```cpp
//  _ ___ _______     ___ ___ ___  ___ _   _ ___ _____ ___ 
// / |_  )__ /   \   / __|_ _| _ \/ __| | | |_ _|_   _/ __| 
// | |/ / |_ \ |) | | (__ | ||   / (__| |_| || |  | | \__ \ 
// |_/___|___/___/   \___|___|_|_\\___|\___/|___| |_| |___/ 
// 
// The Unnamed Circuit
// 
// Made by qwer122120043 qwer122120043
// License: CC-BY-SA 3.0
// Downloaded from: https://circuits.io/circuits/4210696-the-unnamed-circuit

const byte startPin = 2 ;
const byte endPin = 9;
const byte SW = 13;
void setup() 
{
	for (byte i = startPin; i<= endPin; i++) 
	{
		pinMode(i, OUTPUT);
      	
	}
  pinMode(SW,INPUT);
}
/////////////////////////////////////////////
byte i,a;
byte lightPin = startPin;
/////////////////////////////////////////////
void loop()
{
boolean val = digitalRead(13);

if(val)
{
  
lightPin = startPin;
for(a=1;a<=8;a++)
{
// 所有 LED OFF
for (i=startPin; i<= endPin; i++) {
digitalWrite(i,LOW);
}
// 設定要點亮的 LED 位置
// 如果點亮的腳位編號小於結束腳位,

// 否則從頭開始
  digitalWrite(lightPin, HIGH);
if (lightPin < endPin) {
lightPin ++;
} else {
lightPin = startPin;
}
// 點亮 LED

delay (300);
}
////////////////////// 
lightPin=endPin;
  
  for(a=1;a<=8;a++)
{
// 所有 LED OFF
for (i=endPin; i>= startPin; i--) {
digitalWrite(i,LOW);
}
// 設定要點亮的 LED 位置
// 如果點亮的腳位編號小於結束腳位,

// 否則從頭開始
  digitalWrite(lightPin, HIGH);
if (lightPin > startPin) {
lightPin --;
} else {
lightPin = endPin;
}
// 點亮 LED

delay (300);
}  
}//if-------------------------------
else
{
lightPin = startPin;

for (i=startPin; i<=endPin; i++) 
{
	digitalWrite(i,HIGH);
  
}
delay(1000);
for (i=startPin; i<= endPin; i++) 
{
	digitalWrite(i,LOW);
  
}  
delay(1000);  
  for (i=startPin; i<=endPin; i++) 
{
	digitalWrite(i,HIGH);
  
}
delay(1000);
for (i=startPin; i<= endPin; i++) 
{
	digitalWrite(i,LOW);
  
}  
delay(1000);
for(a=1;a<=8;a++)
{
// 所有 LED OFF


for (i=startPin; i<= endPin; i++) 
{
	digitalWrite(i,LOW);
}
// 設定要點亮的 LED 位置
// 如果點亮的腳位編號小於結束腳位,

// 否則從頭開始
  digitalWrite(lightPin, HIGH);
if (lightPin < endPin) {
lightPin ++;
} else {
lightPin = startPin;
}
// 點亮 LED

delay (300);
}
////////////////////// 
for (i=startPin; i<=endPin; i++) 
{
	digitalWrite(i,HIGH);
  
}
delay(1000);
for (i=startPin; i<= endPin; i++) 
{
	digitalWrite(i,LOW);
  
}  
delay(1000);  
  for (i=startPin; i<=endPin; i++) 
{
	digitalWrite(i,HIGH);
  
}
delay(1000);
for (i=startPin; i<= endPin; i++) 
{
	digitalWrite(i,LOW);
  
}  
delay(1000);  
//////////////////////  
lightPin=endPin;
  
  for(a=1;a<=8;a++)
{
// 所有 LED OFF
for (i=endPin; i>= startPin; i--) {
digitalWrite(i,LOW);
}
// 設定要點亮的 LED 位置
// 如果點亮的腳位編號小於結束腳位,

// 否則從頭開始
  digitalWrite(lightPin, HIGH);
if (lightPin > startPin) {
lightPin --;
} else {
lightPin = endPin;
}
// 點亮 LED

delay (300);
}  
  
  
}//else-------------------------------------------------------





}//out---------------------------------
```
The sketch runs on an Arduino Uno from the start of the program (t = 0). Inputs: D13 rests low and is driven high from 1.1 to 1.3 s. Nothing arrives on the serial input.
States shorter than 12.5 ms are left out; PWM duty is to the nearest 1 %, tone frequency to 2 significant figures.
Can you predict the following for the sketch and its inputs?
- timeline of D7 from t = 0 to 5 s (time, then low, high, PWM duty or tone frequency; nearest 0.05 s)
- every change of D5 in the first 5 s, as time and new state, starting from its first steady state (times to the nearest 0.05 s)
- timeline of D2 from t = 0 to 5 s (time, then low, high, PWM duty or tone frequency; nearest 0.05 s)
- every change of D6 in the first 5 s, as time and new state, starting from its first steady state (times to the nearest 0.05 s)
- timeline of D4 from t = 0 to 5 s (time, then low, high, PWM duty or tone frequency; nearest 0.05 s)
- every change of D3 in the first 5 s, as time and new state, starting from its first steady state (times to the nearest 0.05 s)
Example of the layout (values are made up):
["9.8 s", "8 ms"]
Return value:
["0 s high; 1 s low; 2 s high; 3 s low", "0 s high; 1 s low; 2 s high; 3 s low; 4.9 s high", "0 s high; 1 s low; 2 s high; 3 s low; 4 s high; 4.3 s low", "0 s high; 1 s low; 2 s high; 3 s low", "0 s high; 1 s low; 2 s high; 3 s low; 4.6 s high; 4.9 s low", "0 s high; 1 s low; 2 s high; 3 s low; 4.3 s high; 4.6 s low"]
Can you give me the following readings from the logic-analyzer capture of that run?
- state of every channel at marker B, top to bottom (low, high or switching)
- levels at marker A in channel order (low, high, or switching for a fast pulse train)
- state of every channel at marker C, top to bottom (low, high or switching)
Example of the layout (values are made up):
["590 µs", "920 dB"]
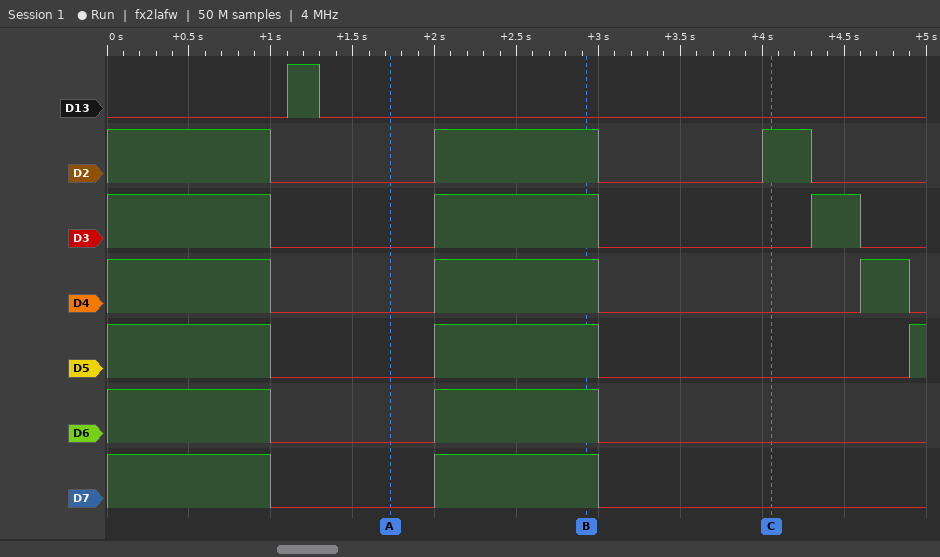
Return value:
["D13 low, D2 high, D3 high, D4 high, D5 high, D6 high, D7 high", "D13 low, D2 low, D3 low, D4 low, D5 low, D6 low, D7 low", "D13 low, D2 high, D3 low, D4 low, D5 low, D6 low, D7 low"]
